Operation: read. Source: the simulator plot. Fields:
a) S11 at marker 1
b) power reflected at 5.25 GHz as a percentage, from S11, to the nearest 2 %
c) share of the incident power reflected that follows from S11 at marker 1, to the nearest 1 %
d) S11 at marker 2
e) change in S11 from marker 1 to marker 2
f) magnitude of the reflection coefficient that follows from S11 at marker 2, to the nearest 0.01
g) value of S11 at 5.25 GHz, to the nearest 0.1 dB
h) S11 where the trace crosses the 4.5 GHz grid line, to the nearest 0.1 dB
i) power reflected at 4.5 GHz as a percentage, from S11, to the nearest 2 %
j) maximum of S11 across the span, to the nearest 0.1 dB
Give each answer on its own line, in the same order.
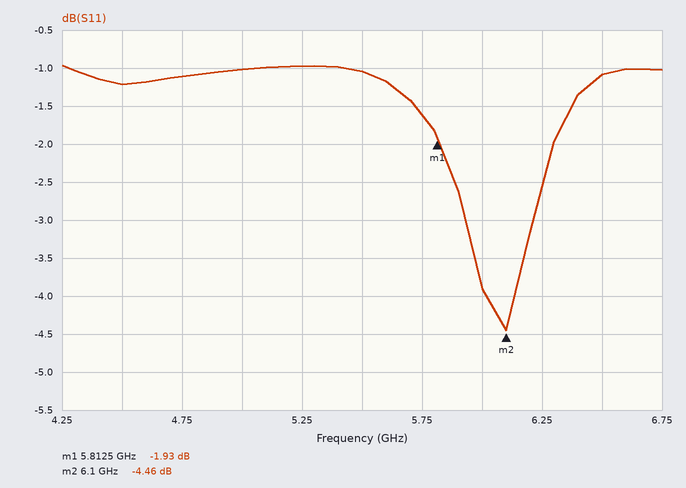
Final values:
-1.93 dB
80 %
64 %
-4.46 dB
-2.53 dB
0.60
-1.0 dB
-1.2 dB
76 %
-1.0 dB
